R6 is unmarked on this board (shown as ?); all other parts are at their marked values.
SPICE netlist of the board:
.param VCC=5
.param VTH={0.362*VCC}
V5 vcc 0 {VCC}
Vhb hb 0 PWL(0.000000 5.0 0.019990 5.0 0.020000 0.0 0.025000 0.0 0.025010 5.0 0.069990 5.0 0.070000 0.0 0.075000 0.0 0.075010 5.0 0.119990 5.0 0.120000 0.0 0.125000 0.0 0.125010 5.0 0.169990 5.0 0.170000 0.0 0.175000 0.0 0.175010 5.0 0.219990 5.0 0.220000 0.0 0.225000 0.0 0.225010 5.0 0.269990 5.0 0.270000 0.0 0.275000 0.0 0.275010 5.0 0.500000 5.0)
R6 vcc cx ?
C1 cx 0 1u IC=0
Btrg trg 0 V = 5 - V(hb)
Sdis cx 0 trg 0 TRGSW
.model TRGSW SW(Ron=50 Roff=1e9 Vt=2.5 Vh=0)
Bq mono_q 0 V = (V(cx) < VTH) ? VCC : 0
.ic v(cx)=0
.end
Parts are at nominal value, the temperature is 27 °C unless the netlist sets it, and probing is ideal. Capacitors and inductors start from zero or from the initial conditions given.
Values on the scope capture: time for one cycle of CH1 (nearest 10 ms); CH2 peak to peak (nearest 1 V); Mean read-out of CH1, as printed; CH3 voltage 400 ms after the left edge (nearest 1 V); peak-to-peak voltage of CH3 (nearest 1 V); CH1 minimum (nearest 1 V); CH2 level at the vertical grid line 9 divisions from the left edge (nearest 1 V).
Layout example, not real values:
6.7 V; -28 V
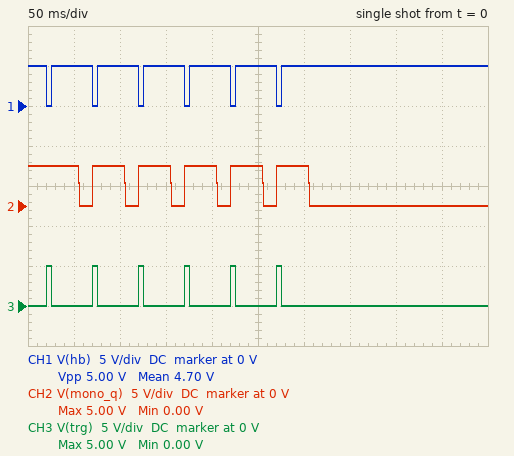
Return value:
50 ms; 5 V; 4.70 V; 0 V; 5 V; 0 V; 0 V
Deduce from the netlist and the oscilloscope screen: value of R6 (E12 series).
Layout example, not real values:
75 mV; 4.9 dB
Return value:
68 kΩ
